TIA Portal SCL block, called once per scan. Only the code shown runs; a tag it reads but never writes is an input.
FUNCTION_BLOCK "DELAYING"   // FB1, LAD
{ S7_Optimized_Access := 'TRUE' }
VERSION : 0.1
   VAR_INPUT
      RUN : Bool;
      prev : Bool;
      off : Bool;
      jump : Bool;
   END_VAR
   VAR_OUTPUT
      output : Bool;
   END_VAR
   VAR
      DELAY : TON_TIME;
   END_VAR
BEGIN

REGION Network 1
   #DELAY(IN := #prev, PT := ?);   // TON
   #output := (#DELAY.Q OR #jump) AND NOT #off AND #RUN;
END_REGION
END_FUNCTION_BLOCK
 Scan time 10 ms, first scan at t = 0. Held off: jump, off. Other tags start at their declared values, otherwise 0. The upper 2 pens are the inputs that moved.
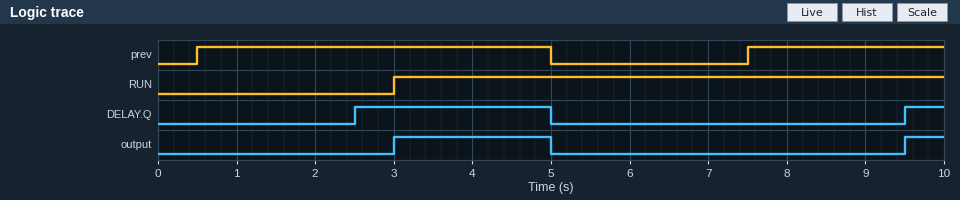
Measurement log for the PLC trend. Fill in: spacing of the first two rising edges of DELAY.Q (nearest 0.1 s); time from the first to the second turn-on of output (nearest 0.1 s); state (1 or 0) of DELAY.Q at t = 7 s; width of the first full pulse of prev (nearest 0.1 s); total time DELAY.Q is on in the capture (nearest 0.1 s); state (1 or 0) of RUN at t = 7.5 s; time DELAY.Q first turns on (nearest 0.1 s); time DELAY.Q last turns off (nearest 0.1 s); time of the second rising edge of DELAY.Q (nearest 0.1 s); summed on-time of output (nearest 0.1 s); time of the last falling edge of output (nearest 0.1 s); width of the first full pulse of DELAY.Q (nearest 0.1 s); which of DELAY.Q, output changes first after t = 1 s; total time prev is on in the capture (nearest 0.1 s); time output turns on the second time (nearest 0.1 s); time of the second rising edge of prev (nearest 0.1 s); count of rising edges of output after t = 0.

7.0 s
6.5 s
0
4.5 s
3.0 s
1
2.5 s
5.0 s
9.5 s
2.5 s
5.0 s
2.5 s
DELAY.Q
7.0 s
9.5 s
7.5 s
2
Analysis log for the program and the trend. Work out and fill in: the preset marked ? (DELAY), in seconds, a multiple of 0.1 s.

2.0 s
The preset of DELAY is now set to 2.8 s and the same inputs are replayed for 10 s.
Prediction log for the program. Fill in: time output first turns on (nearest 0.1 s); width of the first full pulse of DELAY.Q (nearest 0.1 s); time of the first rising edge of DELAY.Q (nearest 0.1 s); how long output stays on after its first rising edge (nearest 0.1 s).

3.3 s
1.7 s
3.3 s
1.7 s
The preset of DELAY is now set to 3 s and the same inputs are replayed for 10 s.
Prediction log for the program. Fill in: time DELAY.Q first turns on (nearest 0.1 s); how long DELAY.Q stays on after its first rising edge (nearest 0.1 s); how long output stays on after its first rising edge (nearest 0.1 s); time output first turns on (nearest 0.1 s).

3.5 s
1.5 s
1.5 s
3.5 s
